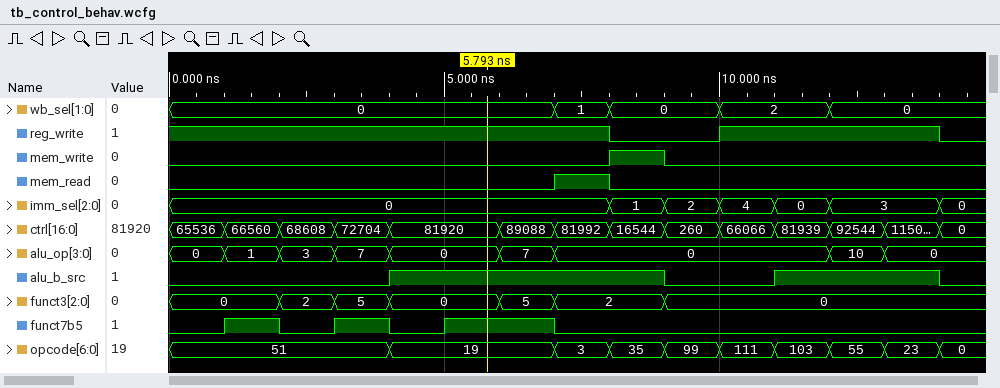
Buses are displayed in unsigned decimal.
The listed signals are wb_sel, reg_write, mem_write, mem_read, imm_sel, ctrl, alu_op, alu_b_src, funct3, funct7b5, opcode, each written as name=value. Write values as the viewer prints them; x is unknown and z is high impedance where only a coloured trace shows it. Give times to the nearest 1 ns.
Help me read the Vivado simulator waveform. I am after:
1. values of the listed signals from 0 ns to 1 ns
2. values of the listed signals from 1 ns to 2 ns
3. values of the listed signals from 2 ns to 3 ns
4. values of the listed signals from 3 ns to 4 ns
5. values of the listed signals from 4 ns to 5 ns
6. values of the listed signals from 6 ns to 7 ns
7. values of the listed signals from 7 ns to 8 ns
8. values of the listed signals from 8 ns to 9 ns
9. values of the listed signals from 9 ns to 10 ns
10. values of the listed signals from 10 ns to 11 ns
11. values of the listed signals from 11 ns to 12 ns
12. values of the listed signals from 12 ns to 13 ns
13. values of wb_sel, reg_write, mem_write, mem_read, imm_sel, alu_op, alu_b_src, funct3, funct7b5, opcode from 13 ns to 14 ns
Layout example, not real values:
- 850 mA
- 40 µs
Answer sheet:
- wb_sel=0, reg_write=1, mem_write=0, mem_read=0, imm_sel=0, ctrl=65536, alu_op=0, alu_b_src=0, funct3=0, funct7b5=0, opcode=51
- wb_sel=0, reg_write=1, mem_write=0, mem_read=0, imm_sel=0, ctrl=66560, alu_op=1, alu_b_src=0, funct3=0, funct7b5=1, opcode=51
- wb_sel=0, reg_write=1, mem_write=0, mem_read=0, imm_sel=0, ctrl=68608, alu_op=3, alu_b_src=0, funct3=2, funct7b5=0, opcode=51
- wb_sel=0, reg_write=1, mem_write=0, mem_read=0, imm_sel=0, ctrl=72704, alu_op=7, alu_b_src=0, funct3=5, funct7b5=1, opcode=51
- wb_sel=0, reg_write=1, mem_write=0, mem_read=0, imm_sel=0, ctrl=81920, alu_op=0, alu_b_src=1, funct3=0, funct7b5=0, opcode=19
- wb_sel=0, reg_write=1, mem_write=0, mem_read=0, imm_sel=0, ctrl=89088, alu_op=7, alu_b_src=1, funct3=5, funct7b5=1, opcode=19
- wb_sel=1, reg_write=1, mem_write=0, mem_read=1, imm_sel=0, ctrl=81992, alu_op=0, alu_b_src=1, funct3=2, funct7b5=0, opcode=3
- wb_sel=0, reg_write=0, mem_write=1, mem_read=0, imm_sel=1, ctrl=16544, alu_op=0, alu_b_src=1, funct3=2, funct7b5=0, opcode=35
- wb_sel=0, reg_write=0, mem_write=0, mem_read=0, imm_sel=2, ctrl=260, alu_op=0, alu_b_src=0, funct3=0, funct7b5=0, opcode=99
- wb_sel=2, reg_write=1, mem_write=0, mem_read=0, imm_sel=4, ctrl=66066, alu_op=0, alu_b_src=0, funct3=0, funct7b5=0, opcode=111
- wb_sel=2, reg_write=1, mem_write=0, mem_read=0, imm_sel=0, ctrl=81939, alu_op=0, alu_b_src=1, funct3=0, funct7b5=0, opcode=103
- wb_sel=0, reg_write=1, mem_write=0, mem_read=0, imm_sel=3, ctrl=92544, alu_op=10, alu_b_src=1, funct3=0, funct7b5=0, opcode=55
- wb_sel=0, reg_write=1, mem_write=0, mem_read=0, imm_sel=3, alu_op=0, alu_b_src=1, funct3=0, funct7b5=0, opcode=23
